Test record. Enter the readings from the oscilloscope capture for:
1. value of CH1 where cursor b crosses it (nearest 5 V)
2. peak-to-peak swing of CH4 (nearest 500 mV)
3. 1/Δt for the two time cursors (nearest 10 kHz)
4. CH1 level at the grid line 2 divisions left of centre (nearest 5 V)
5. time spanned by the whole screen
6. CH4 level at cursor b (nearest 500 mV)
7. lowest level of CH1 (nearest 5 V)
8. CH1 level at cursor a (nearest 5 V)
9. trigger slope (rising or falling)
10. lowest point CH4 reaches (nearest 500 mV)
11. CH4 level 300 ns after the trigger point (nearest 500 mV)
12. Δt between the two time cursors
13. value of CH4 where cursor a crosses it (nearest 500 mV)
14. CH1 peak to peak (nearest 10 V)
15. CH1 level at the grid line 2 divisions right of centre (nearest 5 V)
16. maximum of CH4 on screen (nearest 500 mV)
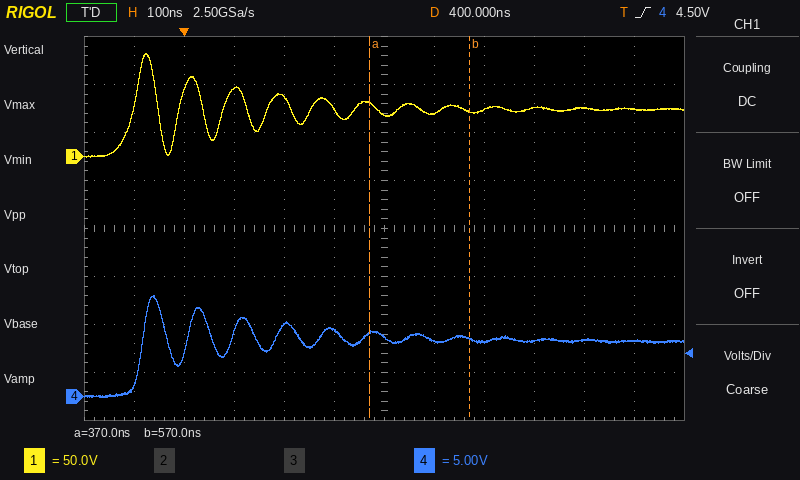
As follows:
45 V
10.5 V
5.00 MHz
60 V
1.2 µs
6.0 V
0 V
55 V
rising
0.0 V
7.0 V
200 ns
6.5 V
110 V
50 V
10.5 V
